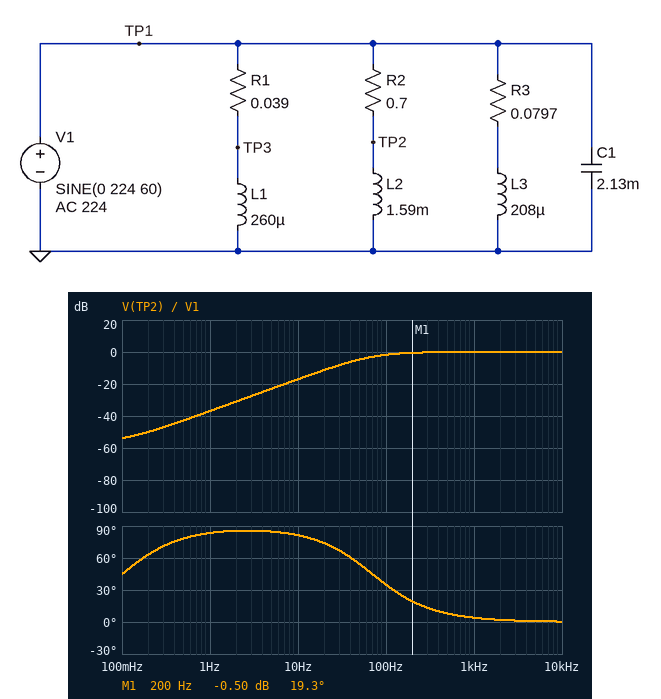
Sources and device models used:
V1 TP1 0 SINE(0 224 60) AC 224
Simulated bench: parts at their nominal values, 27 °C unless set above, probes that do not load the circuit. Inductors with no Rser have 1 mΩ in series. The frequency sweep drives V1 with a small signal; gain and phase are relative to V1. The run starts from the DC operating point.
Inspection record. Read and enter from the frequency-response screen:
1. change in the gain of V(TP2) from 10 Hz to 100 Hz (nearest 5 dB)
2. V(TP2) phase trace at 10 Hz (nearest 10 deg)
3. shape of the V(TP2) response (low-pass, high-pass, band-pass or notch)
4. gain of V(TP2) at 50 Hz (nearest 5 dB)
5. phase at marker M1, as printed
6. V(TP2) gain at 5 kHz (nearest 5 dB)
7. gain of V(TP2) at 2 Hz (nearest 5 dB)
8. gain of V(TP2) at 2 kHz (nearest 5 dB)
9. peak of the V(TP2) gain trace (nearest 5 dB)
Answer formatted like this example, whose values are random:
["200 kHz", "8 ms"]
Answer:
["15 dB", "80 deg", "high-pass", "-5 dB", "19.3 deg", "0 dB", "-30 dB", "0 dB", "0 dB"]
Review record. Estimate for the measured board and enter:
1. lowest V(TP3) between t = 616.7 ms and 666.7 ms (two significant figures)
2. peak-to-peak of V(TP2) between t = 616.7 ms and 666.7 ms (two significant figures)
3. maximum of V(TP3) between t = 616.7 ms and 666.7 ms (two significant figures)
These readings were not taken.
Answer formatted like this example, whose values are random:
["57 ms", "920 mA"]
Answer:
["-210 V", "290 V", "210 V"]
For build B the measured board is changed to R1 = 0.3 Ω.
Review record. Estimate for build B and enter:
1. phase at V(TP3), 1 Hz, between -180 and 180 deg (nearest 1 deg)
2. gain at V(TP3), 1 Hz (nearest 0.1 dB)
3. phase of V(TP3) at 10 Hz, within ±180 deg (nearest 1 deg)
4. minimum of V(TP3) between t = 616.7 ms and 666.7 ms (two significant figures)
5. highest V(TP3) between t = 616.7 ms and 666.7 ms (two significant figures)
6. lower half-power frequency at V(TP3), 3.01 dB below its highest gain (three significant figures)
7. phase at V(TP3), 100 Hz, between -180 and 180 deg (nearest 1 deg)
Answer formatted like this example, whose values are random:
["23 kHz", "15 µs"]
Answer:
["58 deg", "-43.9 dB", "83 deg", "-69 V", "69 V", "184 Hz", "61 deg"]
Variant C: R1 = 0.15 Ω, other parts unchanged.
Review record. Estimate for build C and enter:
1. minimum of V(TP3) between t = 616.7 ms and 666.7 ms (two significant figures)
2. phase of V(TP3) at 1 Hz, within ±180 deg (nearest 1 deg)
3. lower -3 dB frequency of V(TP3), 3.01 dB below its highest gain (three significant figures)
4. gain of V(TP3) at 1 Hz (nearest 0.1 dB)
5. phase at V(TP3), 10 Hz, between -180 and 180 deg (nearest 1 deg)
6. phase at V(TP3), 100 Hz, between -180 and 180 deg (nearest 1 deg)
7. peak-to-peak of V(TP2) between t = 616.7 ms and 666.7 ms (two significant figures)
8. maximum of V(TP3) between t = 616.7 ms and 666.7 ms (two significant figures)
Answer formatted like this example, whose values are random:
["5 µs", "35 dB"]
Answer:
["-120 V", "58 deg", "92.4 Hz", "-37.9 dB", "80 deg", "42 deg", "290 V", "120 V"]
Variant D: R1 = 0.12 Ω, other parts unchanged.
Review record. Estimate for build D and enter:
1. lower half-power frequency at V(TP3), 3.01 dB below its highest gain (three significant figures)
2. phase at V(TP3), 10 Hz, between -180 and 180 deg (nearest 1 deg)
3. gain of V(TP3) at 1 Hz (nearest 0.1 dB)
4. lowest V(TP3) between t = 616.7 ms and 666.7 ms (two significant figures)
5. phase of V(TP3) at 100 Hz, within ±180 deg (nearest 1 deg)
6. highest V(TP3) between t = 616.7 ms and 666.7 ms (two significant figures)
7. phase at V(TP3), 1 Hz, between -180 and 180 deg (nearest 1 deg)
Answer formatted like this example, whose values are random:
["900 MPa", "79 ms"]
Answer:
["74.1 Hz", "79 deg", "-36.0 dB", "-140 V", "36 deg", "140 V", "58 deg"]
